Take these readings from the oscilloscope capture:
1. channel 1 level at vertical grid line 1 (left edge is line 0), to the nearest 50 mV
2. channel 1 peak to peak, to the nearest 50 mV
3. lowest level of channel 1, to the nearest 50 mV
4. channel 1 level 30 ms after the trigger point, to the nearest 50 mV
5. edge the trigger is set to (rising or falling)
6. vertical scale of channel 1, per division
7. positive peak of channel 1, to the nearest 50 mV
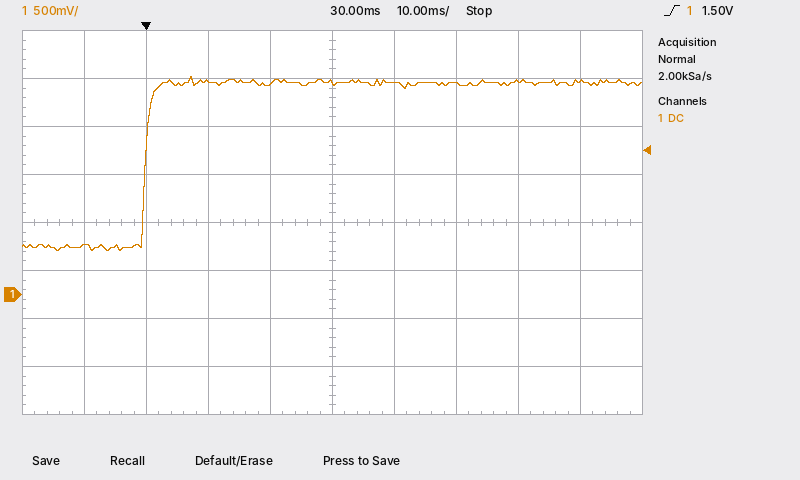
500 mV
1.80 V
450 mV
2.20 V
rising
500 mV
2.25 V
